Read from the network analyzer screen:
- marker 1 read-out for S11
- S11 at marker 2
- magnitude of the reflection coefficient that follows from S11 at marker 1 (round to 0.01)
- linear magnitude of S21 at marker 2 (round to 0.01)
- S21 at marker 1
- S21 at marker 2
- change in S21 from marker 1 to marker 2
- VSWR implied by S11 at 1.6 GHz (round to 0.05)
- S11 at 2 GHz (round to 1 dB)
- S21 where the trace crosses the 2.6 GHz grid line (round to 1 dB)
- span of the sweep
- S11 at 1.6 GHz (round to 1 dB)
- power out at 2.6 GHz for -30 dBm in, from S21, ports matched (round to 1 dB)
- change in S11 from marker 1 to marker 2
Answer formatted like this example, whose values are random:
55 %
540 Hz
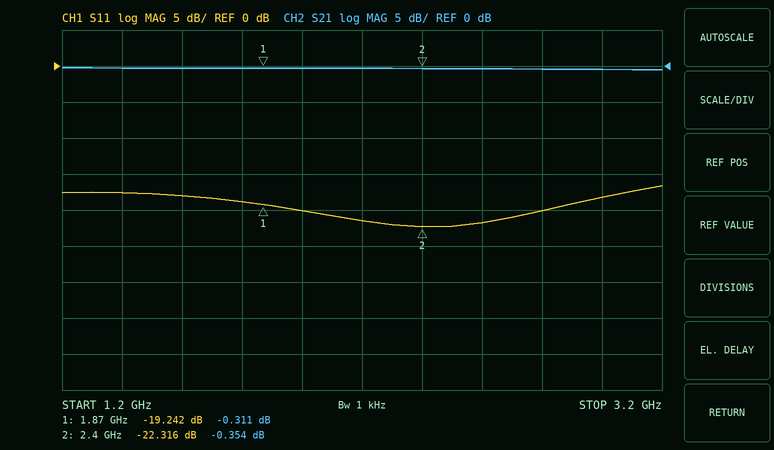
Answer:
-19.242 dB
-22.316 dB
0.11
0.96
-0.311 dB
-0.354 dB
-0.043 dB
1.30
-20 dB
0 dB
2 GHz
-18 dB
-30 dBm
-3.074 dB
